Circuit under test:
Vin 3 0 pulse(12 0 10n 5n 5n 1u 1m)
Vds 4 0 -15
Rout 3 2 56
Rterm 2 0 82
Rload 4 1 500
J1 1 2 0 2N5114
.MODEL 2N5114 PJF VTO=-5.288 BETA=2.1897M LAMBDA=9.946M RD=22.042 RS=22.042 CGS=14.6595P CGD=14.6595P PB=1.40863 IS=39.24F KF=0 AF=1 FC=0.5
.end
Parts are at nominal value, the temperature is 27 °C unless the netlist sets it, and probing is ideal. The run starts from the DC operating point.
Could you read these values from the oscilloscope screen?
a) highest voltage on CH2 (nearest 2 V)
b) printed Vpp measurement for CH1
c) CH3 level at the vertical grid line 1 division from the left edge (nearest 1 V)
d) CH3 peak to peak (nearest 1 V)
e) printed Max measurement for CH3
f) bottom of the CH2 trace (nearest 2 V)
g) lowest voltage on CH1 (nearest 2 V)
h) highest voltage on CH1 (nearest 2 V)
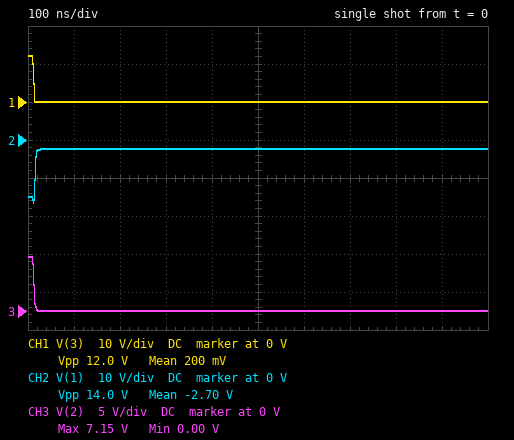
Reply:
-2 V
12.0 V
0 V
7 V
7.15 V
-16 V
0 V
12 V
